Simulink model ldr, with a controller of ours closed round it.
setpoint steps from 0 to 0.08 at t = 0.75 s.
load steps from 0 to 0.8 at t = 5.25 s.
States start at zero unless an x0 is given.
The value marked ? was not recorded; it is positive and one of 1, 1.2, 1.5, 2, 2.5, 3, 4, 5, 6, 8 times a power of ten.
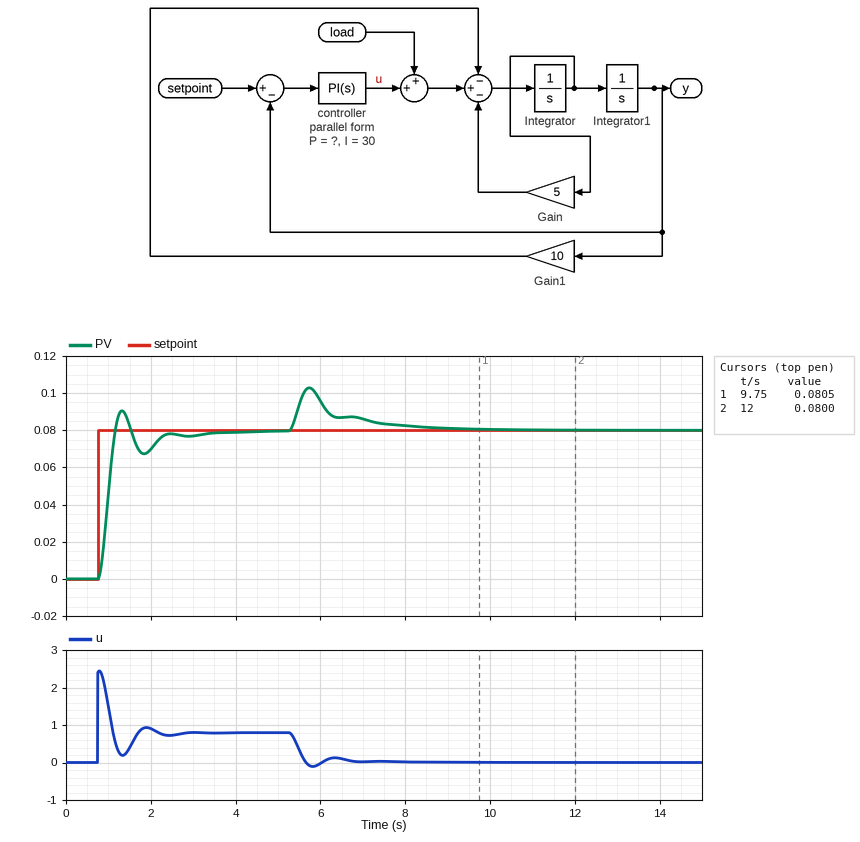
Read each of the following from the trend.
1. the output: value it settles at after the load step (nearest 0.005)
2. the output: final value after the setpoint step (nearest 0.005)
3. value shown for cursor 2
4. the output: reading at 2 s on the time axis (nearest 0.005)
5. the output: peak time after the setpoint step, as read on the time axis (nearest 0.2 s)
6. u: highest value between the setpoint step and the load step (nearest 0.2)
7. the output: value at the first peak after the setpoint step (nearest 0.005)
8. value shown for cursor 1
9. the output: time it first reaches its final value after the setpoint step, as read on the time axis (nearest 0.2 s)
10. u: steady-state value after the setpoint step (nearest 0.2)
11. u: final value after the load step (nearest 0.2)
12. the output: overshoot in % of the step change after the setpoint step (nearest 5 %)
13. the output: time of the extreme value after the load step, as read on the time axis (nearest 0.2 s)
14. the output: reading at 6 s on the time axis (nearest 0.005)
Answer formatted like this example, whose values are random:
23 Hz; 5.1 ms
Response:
0.080; 0.080; 0.0800; 0.070; 1.4 s; 2.4; 0.090; 0.0805; 1.2 s; 0.8; 0.0; 15 %; 5.8 s; 0.095
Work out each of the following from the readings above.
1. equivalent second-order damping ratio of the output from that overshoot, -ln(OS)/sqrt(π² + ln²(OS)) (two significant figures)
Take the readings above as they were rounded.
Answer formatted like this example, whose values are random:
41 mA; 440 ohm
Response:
0.52
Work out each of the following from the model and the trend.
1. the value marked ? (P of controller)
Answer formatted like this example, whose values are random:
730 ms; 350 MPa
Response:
30
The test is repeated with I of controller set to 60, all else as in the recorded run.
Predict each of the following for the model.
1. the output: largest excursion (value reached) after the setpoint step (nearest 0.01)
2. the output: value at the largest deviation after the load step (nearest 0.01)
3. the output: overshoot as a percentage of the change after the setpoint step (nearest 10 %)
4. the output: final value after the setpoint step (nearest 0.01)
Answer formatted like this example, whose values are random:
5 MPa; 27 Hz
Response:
0.10; 0.10; 30 %; 0.08
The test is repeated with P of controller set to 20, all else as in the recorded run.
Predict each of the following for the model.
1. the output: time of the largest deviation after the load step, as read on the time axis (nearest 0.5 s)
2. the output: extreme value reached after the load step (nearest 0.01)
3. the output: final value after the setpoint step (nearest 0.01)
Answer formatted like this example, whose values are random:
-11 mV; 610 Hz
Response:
6.0 s; 0.11; 0.08
